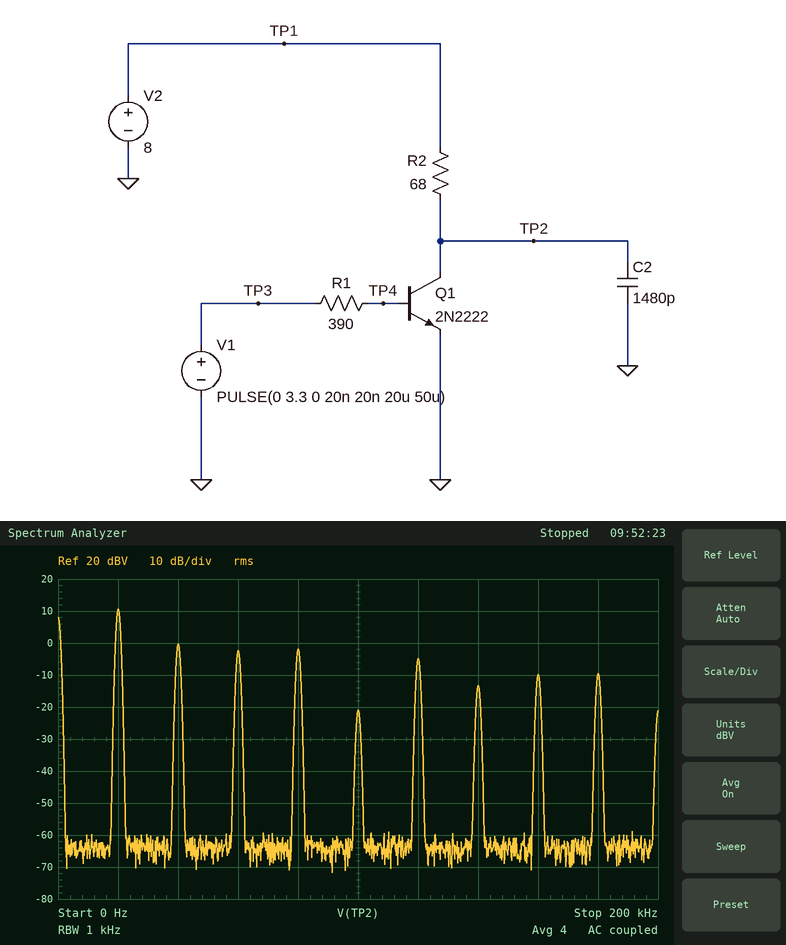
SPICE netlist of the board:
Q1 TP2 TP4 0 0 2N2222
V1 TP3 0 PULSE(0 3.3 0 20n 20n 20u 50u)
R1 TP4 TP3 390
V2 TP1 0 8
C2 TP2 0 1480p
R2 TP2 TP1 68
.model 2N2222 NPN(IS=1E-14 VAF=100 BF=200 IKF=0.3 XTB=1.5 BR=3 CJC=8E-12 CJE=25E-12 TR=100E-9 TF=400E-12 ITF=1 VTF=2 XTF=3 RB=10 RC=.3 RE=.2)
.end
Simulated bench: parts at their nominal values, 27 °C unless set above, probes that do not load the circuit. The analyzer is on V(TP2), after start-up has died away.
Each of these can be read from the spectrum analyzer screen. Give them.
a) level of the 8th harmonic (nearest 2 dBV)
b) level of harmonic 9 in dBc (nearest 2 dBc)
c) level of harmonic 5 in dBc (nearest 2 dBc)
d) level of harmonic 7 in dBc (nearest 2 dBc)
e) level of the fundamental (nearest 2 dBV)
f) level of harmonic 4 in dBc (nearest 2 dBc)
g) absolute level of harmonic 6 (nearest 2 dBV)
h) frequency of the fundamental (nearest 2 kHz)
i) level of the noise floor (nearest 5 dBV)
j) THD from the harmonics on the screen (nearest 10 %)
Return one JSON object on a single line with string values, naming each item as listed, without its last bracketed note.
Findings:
{"level of the 8th harmonic": "-10 dBV", "level of harmonic 9 in dBc": "-20 dBc", "level of harmonic 5 in dBc": "-32 dBc", "level of harmonic 7 in dBc": "-24 dBc", "level of the fundamental": "10 dBV", "level of harmonic 4 in dBc": "-12 dBc", "absolute level of harmonic 6": "-4 dBV", "frequency of the fundamental": "20 kHz", "level of the noise floor": "-65 dBV", "THD from the harmonics on the screen": "50 %"}
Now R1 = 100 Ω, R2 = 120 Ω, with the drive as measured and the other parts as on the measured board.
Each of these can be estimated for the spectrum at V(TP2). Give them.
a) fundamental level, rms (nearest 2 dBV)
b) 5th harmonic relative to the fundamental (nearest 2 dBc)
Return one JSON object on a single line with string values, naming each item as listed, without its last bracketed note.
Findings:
{"fundamental level, rms": "10 dBV", "5th harmonic relative to the fundamental": "-28 dBc"}
